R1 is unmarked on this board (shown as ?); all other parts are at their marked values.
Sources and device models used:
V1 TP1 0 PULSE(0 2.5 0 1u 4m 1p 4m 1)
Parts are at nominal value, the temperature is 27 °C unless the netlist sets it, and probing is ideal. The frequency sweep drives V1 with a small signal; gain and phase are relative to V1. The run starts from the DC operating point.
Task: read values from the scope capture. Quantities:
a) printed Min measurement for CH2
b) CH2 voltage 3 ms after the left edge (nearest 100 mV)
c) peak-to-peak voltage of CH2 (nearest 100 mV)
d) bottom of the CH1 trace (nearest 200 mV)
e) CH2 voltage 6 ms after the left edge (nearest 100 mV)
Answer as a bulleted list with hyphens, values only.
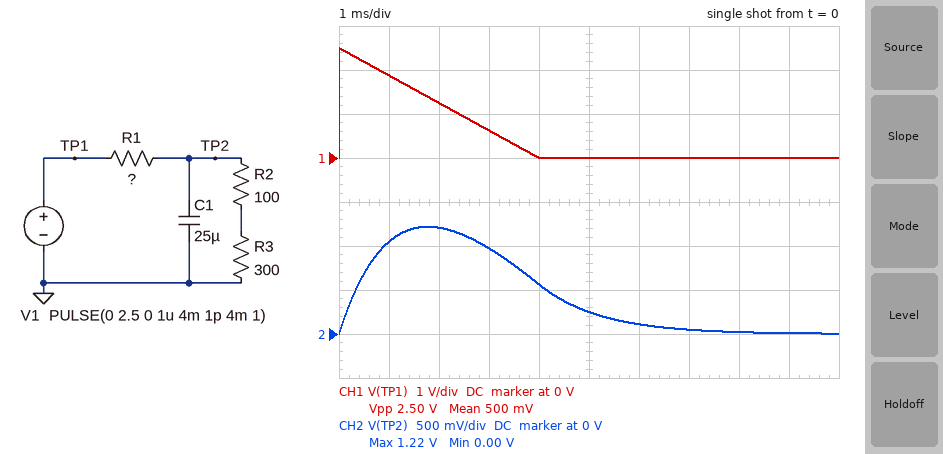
- 0.00 V
- 1.0 V
- 1.2 V
- 0 V
- 100 mV
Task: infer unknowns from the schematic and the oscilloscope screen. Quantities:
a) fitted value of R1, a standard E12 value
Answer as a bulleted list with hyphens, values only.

- 56 Ω
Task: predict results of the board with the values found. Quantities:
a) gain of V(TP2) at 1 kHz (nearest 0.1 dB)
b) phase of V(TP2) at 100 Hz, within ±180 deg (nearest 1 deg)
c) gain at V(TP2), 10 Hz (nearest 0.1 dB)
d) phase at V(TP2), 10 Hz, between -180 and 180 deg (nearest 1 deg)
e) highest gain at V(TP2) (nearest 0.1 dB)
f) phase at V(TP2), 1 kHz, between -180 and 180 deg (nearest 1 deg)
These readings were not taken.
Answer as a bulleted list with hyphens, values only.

- -19.0 dB
- -38 deg
- -1.2 dB
- -4 deg
- -1.1 dB
- -83 deg
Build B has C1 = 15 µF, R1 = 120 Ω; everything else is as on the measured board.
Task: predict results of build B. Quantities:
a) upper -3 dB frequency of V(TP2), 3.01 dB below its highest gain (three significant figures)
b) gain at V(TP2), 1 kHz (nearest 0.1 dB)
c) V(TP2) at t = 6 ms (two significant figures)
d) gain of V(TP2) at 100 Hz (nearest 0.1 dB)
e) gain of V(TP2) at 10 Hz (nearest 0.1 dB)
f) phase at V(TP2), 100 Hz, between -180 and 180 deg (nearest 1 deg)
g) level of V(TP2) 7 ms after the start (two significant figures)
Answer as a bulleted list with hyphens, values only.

- 115 Hz
- -21.1 dB
- 120 mV
- -4.7 dB
- -2.3 dB
- -41 deg
- 60 mV
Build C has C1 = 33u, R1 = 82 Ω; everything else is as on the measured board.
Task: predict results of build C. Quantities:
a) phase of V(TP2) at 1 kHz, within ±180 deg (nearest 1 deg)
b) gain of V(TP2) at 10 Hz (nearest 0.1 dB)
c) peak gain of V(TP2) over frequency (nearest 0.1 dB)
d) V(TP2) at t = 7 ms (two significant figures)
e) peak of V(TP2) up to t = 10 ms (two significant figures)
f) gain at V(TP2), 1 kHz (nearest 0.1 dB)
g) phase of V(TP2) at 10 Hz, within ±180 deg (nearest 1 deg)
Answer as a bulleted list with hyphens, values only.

- -86 deg
- -1.7 dB
- -1.6 dB
- 160 mV
- 880 mV
- -24.6 dB
- -8 deg
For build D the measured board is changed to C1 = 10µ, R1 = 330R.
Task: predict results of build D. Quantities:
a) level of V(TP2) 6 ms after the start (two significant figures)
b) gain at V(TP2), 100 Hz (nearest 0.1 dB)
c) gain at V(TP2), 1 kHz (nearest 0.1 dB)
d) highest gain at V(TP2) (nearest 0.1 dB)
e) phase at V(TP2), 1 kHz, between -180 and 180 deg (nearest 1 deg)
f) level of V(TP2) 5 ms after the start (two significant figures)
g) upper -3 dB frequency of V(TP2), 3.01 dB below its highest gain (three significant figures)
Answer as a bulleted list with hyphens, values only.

- 130 mV
- -8.8 dB
- -26.4 dB
- -5.2 dB
- -85 deg
- 230 mV
- 88.0 Hz
